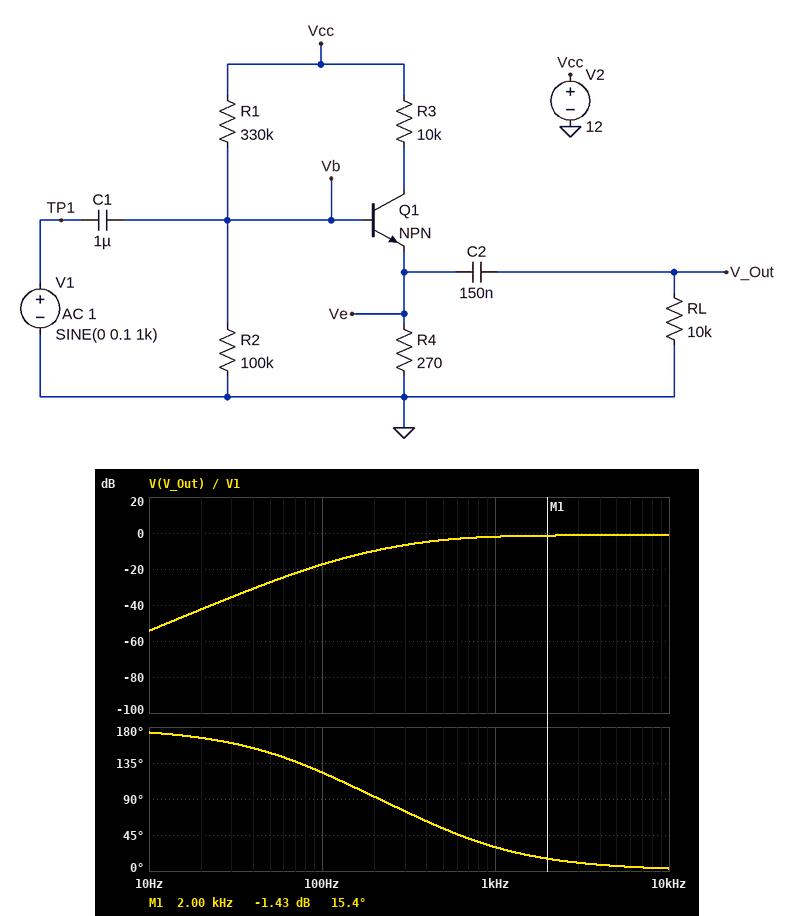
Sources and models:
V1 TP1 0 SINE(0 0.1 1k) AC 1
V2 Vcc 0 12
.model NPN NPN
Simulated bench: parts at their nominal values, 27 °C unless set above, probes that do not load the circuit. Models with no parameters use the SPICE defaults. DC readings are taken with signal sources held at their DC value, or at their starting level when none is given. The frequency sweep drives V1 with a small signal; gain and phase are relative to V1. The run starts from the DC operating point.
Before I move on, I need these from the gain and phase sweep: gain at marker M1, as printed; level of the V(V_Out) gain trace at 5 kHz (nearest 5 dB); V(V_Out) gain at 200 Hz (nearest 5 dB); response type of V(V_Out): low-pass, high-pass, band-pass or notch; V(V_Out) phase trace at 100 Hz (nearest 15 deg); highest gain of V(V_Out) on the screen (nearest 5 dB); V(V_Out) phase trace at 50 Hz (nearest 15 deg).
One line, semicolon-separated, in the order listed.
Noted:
-1.43 dB; 0 dB; -10 dB; high-pass; 120 deg; 0 dB; 150 deg
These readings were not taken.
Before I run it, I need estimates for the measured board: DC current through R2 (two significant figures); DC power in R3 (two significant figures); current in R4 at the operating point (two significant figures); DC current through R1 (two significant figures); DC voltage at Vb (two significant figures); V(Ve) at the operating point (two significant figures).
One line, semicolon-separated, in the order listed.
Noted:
11 µA; 13 mW; 1.2 mA; 33 µA; 1.1 V; 320 mV
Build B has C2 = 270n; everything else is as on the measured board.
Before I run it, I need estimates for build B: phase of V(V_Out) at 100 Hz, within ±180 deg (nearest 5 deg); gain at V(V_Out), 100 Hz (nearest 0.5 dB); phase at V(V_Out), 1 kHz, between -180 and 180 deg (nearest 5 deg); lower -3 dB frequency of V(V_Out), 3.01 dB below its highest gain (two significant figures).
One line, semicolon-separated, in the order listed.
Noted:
105 deg; -15.5 dB; 25 deg; 450 Hz
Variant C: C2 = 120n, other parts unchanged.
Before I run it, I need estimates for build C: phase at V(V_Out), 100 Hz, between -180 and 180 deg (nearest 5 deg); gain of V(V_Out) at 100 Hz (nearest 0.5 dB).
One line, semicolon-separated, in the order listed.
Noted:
130 deg; -18.5 dB
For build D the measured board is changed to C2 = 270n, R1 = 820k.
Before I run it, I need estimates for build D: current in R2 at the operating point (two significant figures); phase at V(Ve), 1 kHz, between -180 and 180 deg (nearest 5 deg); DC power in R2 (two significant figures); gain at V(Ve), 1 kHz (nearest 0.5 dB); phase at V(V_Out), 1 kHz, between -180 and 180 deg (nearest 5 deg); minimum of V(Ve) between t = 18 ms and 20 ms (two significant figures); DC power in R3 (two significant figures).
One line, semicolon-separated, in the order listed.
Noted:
8.8 µA; 0 deg; 7.8 µW; -1.5 dB; 5 deg; 52 mV; 2.2 mW
